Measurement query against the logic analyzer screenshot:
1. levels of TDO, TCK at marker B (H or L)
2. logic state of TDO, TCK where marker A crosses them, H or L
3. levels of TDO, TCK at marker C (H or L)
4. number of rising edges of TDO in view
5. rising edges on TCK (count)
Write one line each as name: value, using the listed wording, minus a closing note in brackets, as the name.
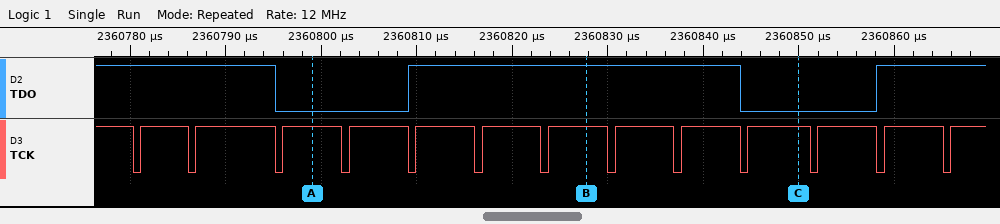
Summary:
levels of TDO, TCK at marker B: TDO=H, TCK=H
logic state of TDO, TCK where marker A crosses them, H or L: TDO=L, TCK=H
levels of TDO, TCK at marker C: TDO=L, TCK=H
number of rising edges of TDO in view: 2
rising edges on TCK: 13
